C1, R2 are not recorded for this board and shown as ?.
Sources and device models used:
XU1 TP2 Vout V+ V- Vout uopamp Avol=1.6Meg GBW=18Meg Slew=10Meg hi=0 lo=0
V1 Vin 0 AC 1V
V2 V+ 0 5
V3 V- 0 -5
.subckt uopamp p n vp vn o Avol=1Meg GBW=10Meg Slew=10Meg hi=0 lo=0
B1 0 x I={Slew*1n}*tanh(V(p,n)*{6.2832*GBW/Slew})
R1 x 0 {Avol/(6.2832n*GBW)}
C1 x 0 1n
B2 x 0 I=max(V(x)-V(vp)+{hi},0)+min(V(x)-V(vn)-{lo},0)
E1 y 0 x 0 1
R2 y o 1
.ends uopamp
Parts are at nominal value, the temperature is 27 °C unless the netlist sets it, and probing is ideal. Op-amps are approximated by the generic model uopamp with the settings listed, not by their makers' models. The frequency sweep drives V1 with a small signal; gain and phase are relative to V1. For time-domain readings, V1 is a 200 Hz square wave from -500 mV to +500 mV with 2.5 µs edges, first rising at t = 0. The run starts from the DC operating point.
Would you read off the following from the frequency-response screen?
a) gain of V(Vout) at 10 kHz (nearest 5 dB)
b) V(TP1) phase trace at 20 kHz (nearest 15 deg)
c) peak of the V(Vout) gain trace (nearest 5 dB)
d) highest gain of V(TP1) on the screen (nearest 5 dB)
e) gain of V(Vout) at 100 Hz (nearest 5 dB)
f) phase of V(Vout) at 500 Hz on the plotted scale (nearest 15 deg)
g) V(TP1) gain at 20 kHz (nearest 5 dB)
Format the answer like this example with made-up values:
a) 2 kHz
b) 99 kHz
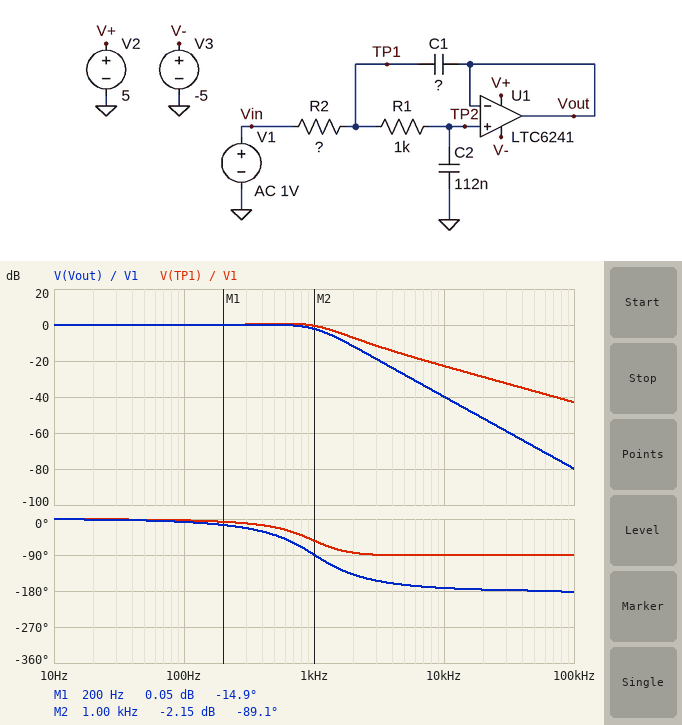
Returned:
a) -40 dB
b) -90 deg
c) 0 dB
d) 0 dB
e) 0 dB
f) -45 deg
g) -30 dB
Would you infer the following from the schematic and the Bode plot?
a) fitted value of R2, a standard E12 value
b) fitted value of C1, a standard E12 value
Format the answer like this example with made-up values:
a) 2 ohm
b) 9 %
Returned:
a) 820 Ω
b) 270 nF
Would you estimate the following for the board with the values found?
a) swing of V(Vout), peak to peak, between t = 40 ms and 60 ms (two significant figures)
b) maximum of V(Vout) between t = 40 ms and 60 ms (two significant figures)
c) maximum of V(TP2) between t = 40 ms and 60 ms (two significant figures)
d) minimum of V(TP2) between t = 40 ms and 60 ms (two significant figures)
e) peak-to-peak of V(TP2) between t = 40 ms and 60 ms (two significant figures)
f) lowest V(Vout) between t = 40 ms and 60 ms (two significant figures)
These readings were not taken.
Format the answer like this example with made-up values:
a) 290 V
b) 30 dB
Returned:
a) 1.1 V
b) 570 mV
c) 570 mV
d) -570 mV
e) 1.1 V
f) -570 mV
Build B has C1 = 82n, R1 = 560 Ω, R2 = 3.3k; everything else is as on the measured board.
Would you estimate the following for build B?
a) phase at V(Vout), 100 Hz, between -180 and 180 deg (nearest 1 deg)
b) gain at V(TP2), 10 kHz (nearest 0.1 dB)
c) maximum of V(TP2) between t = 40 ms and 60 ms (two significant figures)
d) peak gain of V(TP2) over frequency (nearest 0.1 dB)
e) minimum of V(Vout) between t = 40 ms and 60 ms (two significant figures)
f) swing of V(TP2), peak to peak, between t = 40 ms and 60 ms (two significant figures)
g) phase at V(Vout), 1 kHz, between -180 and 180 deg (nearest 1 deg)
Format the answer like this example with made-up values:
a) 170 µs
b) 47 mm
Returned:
a) -15 deg
b) -37.1 dB
c) 500 mV
d) 0 dB
e) -500 mV
f) 1.0 V
g) -83 deg
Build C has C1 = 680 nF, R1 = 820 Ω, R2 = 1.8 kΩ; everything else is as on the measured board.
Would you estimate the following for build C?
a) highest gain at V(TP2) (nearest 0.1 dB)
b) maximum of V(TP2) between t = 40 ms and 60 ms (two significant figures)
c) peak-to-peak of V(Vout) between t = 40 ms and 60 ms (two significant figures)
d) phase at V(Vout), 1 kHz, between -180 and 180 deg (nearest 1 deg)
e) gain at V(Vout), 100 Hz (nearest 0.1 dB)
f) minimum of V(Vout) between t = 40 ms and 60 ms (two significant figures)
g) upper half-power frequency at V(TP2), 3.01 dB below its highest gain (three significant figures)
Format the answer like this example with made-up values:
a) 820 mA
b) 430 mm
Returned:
a) 2.1 dB
b) 710 mV
c) 1.4 V
d) -152 deg
e) 0.2 dB
f) -710 mV
g) 562 Hz
